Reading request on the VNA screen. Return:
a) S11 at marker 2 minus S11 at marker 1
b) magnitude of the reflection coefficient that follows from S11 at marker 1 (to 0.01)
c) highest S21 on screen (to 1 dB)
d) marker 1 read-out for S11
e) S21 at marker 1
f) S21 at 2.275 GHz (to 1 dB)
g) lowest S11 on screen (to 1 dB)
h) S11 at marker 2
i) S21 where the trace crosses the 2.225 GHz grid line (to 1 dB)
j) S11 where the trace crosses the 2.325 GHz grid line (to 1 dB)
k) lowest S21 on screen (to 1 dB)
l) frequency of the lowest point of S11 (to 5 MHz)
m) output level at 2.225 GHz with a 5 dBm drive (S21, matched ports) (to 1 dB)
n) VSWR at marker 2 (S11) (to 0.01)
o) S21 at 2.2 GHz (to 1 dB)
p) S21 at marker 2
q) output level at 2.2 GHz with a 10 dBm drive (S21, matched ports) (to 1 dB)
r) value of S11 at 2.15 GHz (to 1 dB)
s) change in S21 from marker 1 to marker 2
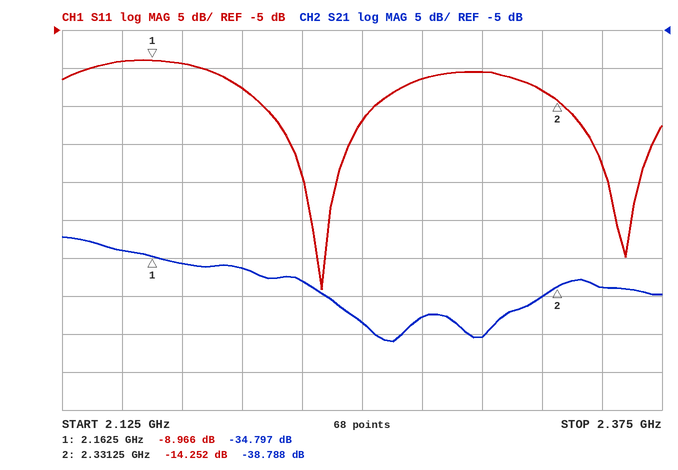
-5.286 dB
0.36
-32 dB
-8.966 dB
-34.797 dB
-43 dB
-39 dB
-14.252 dB
-38 dB
-13 dB
-46 dB
2.235 GHz
-33 dBm
1.48
-36 dB
-38.788 dB
-26 dBm
-9 dB
-3.991 dB
